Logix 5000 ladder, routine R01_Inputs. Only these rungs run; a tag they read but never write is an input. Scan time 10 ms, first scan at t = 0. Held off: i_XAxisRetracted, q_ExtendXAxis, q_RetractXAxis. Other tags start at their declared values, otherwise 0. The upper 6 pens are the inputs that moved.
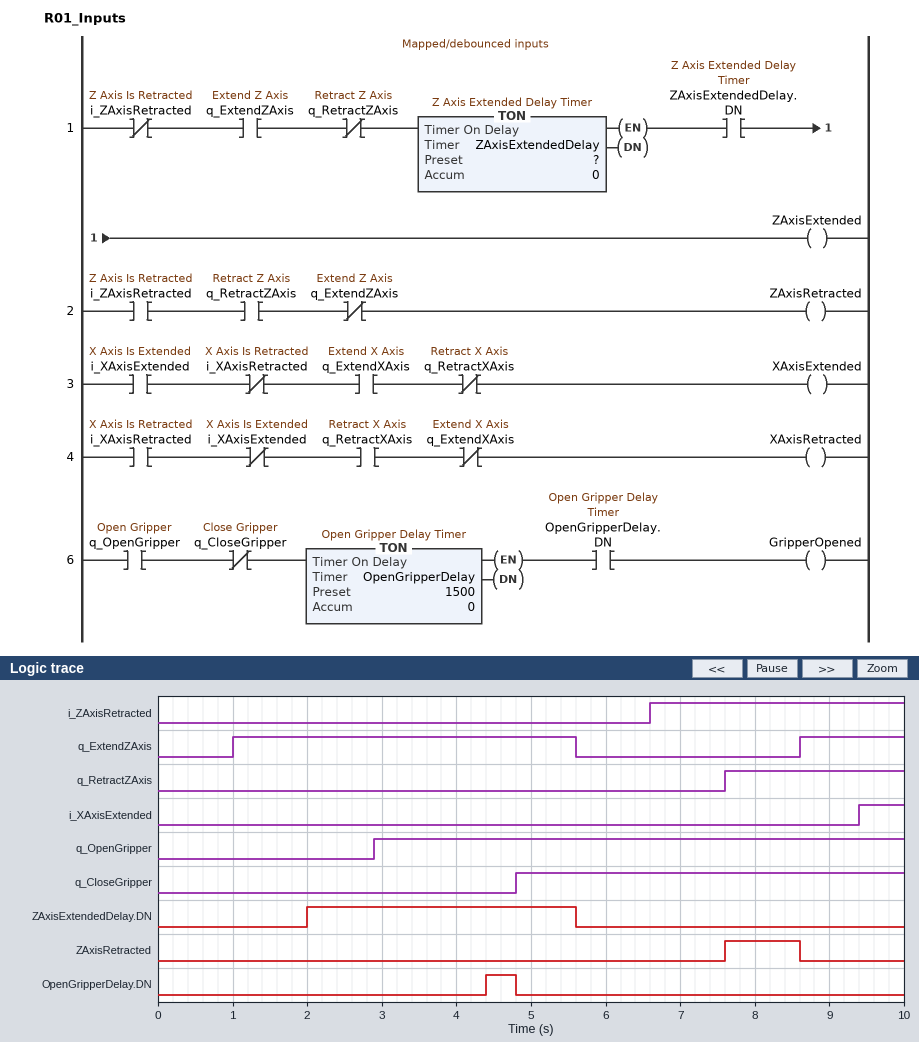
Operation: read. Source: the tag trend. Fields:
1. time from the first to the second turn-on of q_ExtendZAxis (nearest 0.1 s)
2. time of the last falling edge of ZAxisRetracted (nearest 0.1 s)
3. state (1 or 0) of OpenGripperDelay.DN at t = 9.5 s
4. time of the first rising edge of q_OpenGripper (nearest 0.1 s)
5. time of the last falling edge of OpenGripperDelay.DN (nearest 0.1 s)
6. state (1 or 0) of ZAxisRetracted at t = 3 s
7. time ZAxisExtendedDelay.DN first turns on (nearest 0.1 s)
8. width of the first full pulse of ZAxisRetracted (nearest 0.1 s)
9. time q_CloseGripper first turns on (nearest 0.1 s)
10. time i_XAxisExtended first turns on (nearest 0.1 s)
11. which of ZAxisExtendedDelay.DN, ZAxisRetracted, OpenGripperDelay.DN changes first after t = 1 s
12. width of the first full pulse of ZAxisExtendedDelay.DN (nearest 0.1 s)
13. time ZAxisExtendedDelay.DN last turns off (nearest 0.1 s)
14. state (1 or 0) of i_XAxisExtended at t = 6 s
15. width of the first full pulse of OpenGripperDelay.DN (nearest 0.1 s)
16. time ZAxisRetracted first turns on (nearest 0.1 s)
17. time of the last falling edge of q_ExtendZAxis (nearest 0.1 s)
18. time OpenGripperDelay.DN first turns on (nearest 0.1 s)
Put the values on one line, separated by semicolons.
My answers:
7.6 s; 8.6 s; 0; 2.9 s; 4.8 s; 0; 2.0 s; 1.0 s; 4.8 s; 9.4 s; ZAxisExtendedDelay.DN; 3.6 s; 5.6 s; 0; 0.4 s; 7.6 s; 5.6 s; 4.4 s
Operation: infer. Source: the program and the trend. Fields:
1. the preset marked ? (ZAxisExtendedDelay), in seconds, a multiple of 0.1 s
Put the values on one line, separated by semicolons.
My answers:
1.0 s
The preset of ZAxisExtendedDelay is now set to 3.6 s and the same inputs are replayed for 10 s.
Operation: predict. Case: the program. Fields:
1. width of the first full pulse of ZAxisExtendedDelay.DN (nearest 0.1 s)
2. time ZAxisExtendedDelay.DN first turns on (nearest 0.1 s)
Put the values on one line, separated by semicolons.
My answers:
1.0 s; 4.6 s
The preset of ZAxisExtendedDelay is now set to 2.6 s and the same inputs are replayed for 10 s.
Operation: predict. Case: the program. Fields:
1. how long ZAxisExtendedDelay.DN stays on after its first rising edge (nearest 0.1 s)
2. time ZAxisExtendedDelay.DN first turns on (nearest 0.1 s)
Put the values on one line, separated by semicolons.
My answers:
2.0 s; 3.6 s
